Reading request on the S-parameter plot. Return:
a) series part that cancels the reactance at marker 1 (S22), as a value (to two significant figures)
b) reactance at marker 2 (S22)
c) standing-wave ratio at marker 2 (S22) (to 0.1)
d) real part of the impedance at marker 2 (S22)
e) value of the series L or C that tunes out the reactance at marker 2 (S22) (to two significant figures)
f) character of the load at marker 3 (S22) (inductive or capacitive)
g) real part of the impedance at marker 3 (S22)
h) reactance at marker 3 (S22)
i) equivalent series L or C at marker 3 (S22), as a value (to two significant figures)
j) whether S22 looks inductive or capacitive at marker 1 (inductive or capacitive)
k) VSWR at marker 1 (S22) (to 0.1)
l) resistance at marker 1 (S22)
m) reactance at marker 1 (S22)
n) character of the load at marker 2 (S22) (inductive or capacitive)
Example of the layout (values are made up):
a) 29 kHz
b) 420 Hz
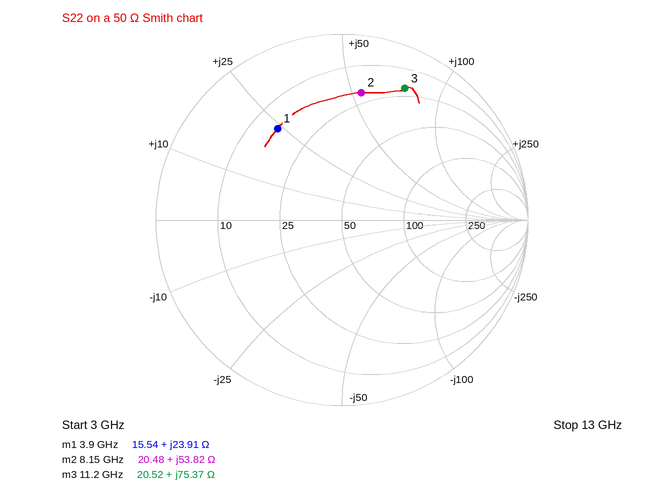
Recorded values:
a) 1.7 pF
b) +53.82 Ω
c) 5.5
d) 20.48 Ω
e) 360 fF
f) inductive
g) 20.52 Ω
h) +75.37 Ω
i) 1.1 nH
j) inductive
k) 4.0
l) 15.54 Ω
m) +23.91 Ω
n) inductive
